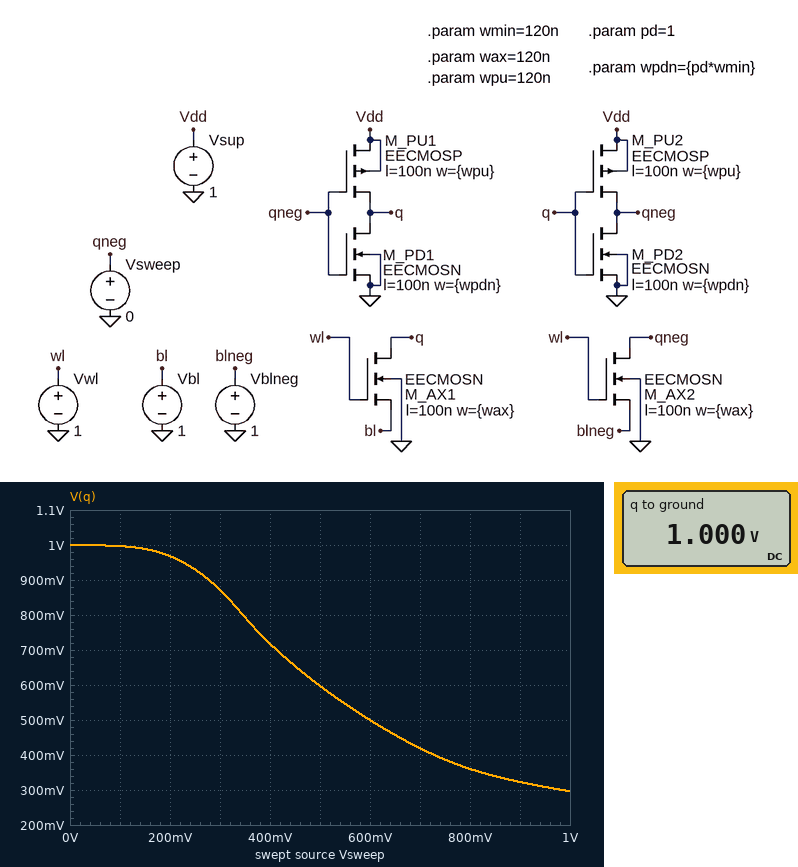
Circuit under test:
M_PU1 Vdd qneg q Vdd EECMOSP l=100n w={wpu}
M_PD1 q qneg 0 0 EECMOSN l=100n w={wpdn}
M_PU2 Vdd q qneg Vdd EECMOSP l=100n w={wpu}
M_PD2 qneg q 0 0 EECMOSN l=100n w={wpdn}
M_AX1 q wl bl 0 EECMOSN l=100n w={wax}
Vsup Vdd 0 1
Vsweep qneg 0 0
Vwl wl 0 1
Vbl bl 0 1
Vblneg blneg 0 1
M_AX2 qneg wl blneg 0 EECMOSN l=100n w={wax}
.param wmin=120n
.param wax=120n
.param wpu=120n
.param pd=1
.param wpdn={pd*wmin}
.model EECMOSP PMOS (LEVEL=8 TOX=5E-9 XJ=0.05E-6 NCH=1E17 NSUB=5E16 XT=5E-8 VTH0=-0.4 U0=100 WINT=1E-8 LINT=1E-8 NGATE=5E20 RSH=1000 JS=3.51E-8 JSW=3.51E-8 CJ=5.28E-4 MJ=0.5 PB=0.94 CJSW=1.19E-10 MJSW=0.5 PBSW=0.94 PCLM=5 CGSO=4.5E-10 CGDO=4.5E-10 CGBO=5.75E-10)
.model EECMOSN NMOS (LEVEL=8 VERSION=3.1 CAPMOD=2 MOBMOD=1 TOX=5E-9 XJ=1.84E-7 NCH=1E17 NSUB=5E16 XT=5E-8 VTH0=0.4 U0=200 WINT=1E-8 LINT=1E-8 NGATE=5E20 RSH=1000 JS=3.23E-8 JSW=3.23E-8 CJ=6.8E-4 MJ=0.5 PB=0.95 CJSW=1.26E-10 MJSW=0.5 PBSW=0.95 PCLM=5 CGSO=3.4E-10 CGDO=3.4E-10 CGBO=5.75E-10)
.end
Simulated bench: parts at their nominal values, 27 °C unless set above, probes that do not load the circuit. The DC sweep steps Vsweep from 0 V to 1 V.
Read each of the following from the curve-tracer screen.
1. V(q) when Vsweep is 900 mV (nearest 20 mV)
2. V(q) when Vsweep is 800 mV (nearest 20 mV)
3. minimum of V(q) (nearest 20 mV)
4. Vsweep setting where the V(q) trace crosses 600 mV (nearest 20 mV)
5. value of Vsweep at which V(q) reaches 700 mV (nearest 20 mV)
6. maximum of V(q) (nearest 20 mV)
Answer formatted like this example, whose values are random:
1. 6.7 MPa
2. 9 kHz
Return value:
1. 320 mV
2. 360 mV
3. 300 mV
4. 500 mV
5. 420 mV
6. 1.00 V
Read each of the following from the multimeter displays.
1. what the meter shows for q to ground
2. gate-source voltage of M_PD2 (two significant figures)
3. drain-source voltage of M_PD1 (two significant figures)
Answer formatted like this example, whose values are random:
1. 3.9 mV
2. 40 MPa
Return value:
1. 1.000 V
2. 1.0 V
3. 1.0 V
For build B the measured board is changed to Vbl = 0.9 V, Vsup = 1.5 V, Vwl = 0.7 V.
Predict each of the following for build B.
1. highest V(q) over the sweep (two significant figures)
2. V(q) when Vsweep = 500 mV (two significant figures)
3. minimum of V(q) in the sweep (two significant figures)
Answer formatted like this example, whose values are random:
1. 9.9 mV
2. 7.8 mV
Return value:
1. 1.5 V
2. 1.1 V
3. 240 mV
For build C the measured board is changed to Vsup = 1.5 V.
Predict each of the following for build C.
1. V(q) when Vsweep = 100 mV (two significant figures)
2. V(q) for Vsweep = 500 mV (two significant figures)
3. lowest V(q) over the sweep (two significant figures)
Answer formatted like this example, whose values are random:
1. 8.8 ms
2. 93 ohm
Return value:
1. 1.5 V
2. 1.1 V
3. 380 mV
